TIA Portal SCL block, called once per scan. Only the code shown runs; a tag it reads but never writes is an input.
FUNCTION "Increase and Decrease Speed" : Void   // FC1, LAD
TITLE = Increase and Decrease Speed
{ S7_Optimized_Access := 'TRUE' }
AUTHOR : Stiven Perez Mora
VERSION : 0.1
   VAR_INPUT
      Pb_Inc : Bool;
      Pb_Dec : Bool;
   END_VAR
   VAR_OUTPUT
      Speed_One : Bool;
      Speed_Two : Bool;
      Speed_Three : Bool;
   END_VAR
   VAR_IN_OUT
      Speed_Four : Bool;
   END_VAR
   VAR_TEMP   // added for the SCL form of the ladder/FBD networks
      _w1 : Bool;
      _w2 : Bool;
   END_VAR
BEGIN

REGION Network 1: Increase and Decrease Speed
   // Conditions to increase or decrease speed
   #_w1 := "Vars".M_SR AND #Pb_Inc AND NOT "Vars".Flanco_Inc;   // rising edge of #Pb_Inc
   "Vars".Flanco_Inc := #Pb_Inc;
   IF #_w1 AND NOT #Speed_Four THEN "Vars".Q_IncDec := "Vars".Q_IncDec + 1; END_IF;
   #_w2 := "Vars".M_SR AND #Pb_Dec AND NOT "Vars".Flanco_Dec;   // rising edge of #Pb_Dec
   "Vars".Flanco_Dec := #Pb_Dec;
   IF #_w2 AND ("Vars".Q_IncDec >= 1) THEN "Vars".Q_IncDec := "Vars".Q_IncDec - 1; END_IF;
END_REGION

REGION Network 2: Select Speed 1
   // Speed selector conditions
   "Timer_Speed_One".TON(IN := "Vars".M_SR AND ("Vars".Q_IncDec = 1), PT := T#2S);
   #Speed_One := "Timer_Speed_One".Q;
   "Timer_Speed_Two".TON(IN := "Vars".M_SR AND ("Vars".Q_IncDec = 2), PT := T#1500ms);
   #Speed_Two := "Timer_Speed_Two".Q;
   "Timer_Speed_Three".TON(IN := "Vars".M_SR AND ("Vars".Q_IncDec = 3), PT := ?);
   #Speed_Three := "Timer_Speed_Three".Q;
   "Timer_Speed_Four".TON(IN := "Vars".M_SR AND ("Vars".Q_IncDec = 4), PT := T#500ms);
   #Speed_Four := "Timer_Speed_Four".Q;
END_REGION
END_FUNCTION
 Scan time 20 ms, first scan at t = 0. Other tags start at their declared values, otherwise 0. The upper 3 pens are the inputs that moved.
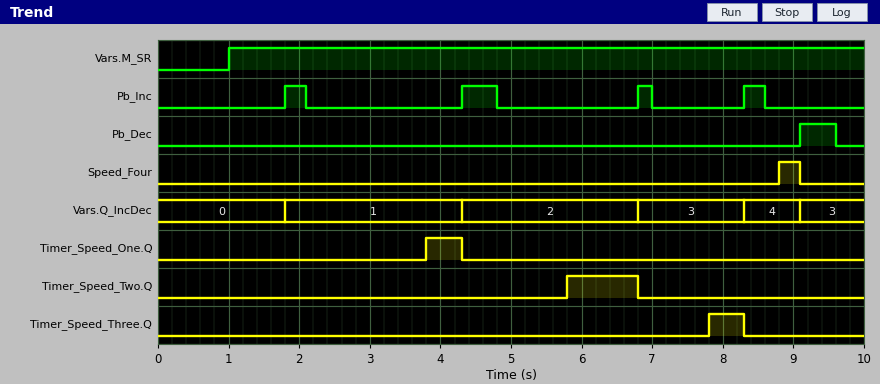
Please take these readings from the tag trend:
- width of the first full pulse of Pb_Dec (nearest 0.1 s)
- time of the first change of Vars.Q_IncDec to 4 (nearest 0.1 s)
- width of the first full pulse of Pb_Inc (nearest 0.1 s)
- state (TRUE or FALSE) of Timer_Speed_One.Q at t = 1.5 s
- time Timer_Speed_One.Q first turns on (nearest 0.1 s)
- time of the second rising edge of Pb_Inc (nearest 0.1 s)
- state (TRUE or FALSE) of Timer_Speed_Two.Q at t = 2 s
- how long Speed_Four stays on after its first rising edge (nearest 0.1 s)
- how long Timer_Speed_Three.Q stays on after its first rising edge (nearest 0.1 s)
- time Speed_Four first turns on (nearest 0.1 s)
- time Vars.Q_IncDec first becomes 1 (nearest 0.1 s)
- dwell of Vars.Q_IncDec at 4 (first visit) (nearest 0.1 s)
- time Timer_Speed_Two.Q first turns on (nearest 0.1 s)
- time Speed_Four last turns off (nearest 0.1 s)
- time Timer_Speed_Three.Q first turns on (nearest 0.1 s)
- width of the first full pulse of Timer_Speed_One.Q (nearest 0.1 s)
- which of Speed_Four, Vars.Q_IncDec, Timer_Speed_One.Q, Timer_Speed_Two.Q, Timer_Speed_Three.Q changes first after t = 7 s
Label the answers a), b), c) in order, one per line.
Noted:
a) 0.5 s
b) 8.3 s
c) 0.3 s
d) FALSE
e) 3.8 s
f) 4.3 s
g) FALSE
h) 0.3 s
i) 0.5 s
j) 8.8 s
k) 1.8 s
l) 0.8 s
m) 5.8 s
n) 9.1 s
o) 7.8 s
p) 0.5 s
q) Timer_Speed_Three.Q
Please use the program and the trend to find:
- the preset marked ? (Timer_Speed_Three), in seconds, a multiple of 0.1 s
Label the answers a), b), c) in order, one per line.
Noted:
a) 1.0 s
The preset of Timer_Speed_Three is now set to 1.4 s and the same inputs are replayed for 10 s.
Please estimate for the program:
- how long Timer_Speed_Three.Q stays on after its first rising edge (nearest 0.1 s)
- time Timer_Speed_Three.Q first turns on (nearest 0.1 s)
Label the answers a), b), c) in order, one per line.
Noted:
a) 0.1 s
b) 8.2 s
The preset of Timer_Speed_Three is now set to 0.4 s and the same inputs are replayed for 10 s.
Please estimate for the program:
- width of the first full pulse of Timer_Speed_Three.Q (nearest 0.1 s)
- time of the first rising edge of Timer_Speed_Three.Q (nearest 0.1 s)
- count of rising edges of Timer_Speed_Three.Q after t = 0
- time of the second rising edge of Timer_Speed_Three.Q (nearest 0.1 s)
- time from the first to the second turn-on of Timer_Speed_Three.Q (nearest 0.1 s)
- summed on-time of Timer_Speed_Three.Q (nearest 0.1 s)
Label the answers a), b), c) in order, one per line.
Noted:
a) 1.1 s
b) 7.2 s
c) 2
d) 9.5 s
e) 2.3 s
f) 1.6 s
